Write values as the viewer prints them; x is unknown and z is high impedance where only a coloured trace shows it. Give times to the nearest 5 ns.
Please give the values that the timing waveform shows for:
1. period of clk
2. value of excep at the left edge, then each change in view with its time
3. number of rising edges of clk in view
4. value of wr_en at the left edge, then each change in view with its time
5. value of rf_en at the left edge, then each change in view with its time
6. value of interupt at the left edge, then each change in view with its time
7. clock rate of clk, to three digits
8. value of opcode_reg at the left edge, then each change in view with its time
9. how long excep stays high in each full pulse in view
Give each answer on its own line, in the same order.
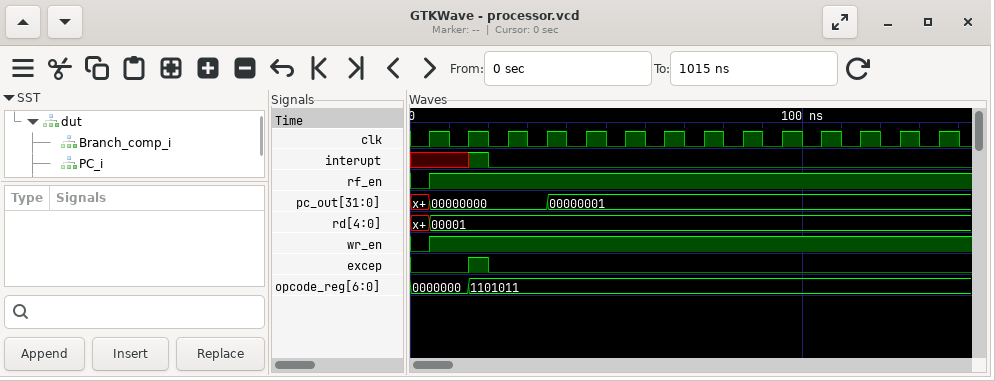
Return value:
10 ns
0, 1 at 15 ns, 0 at 20 ns
14
0, 1 at 5 ns
0, 1 at 5 ns
x, 1 at 15 ns, 0 at 20 ns
100 MHz
0000000, 1101011 at 15 ns
5 ns
